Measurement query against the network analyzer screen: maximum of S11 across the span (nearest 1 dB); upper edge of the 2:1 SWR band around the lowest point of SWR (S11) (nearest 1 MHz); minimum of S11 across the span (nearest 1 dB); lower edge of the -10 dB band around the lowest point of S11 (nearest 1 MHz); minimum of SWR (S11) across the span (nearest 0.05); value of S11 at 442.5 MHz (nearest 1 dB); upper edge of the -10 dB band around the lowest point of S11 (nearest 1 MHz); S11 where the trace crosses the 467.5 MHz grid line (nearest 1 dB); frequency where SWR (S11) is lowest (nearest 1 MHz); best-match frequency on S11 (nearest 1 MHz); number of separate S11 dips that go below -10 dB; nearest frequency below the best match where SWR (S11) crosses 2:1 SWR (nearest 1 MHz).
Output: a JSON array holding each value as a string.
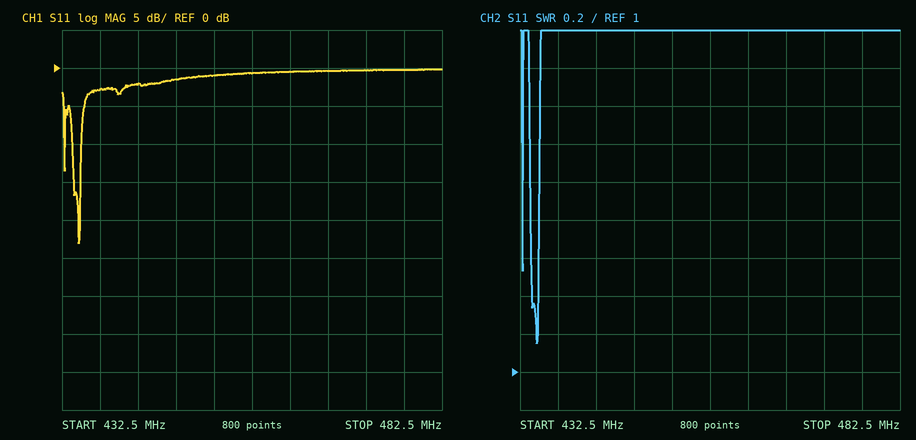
["0 dB", "435 MHz", "-23 dB", "434 MHz", "1.15", "-2 dB", "435 MHz", "0 dB", "435 MHz", "435 MHz", "2", "434 MHz"]
